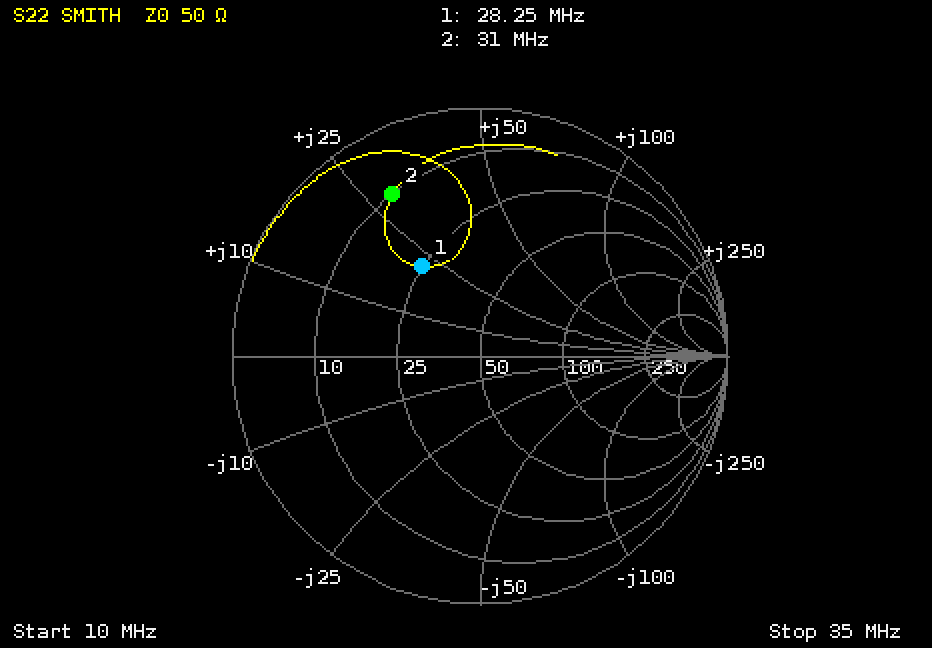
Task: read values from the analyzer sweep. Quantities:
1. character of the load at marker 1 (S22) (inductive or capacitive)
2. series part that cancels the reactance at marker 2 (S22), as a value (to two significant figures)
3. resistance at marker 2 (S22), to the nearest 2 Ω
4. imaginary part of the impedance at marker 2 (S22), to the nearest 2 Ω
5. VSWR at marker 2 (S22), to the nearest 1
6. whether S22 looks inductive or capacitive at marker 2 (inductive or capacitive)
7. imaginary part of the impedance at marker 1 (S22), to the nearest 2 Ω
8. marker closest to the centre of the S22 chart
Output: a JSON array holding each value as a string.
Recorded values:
["inductive", "180 pF", "10 Ω", "+28 Ω", "7", "inductive", "+22 Ω", "marker 1"]
